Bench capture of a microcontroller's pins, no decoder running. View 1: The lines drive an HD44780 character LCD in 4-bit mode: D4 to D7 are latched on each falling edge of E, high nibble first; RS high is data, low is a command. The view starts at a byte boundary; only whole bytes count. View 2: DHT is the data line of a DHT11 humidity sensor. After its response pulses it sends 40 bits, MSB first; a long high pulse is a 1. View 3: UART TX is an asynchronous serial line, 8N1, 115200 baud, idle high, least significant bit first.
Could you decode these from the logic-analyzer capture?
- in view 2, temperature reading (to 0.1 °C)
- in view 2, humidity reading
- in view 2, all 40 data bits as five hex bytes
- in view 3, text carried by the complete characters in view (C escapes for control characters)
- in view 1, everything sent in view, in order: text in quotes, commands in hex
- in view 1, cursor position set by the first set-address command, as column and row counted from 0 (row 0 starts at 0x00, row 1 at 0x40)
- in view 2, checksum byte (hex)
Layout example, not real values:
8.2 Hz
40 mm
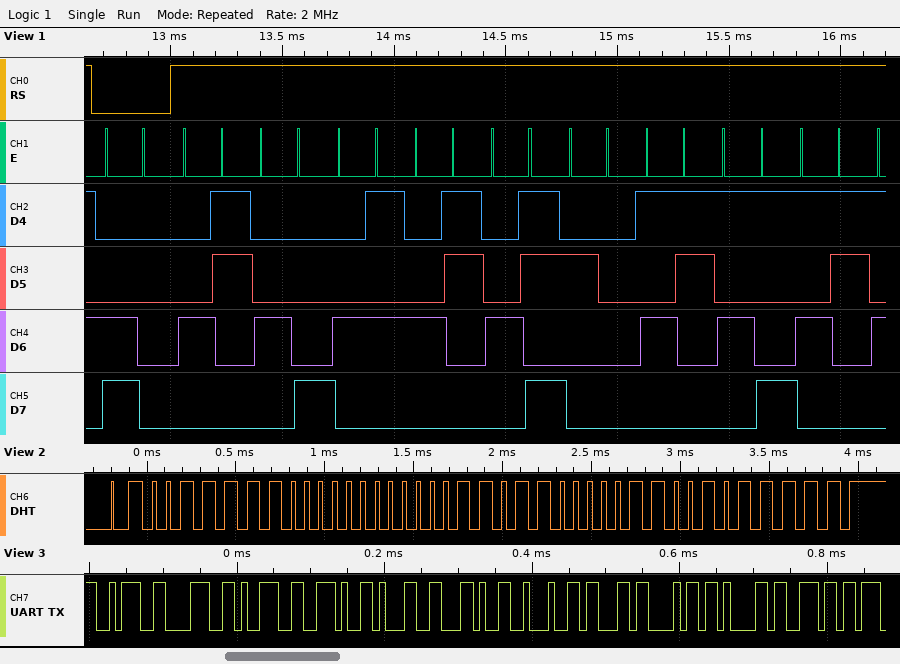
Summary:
27.6 °C
62 %
3E 00 1B 06 5F
":89.1,\"chan"
0xC0 "CHECK SYS"
column 0, row 1
0x5F
